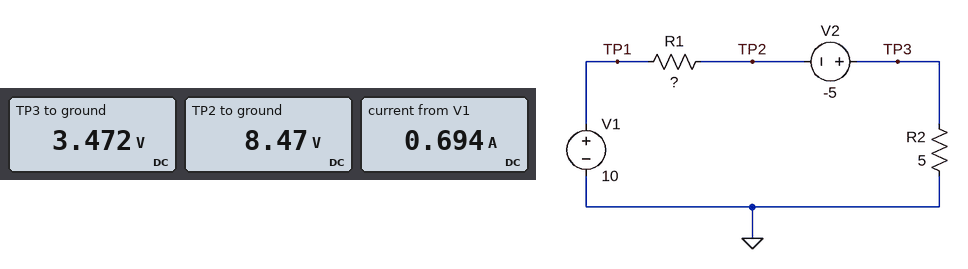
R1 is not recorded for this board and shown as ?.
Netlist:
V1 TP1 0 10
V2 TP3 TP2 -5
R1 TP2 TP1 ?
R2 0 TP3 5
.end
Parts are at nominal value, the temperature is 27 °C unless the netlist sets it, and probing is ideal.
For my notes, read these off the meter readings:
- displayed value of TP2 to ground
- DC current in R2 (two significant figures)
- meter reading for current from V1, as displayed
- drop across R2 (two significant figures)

8.47 V
690 mA
0.694 A
3.5 V
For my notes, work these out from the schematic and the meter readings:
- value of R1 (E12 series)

2.2 Ω
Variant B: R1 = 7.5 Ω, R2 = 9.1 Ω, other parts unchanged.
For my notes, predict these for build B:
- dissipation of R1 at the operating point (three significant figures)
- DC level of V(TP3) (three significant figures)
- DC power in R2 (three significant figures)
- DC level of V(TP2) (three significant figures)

680 mW
2.74 V
826 mW
7.74 V
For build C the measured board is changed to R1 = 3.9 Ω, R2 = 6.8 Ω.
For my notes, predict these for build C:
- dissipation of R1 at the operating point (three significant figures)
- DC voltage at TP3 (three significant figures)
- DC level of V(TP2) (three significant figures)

852 mW
3.18 V
8.18 V
